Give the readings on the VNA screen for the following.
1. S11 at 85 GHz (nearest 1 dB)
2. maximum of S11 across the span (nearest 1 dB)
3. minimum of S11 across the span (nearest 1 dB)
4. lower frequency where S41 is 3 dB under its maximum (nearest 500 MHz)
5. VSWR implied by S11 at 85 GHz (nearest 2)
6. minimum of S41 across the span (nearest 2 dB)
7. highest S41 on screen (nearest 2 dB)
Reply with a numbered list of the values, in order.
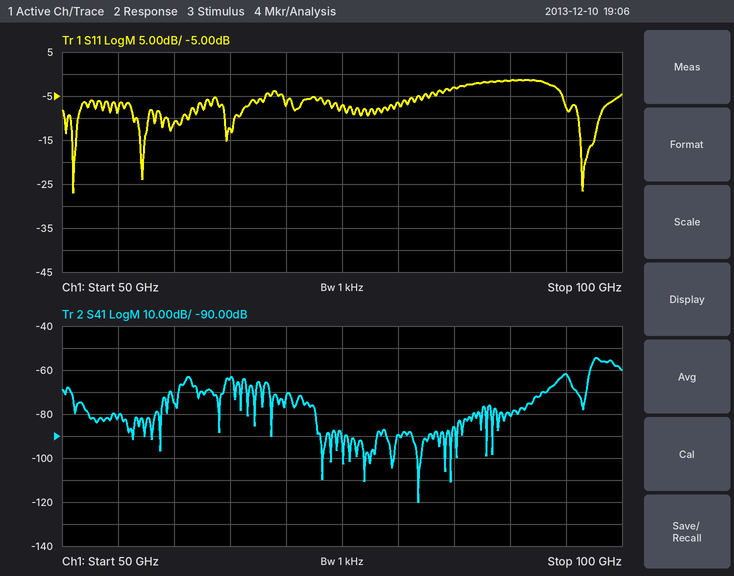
1. -3 dB
2. -1 dB
3. -27 dB
4. 97.5 GHz
5. 6
6. -120 dB
7. -54 dB
